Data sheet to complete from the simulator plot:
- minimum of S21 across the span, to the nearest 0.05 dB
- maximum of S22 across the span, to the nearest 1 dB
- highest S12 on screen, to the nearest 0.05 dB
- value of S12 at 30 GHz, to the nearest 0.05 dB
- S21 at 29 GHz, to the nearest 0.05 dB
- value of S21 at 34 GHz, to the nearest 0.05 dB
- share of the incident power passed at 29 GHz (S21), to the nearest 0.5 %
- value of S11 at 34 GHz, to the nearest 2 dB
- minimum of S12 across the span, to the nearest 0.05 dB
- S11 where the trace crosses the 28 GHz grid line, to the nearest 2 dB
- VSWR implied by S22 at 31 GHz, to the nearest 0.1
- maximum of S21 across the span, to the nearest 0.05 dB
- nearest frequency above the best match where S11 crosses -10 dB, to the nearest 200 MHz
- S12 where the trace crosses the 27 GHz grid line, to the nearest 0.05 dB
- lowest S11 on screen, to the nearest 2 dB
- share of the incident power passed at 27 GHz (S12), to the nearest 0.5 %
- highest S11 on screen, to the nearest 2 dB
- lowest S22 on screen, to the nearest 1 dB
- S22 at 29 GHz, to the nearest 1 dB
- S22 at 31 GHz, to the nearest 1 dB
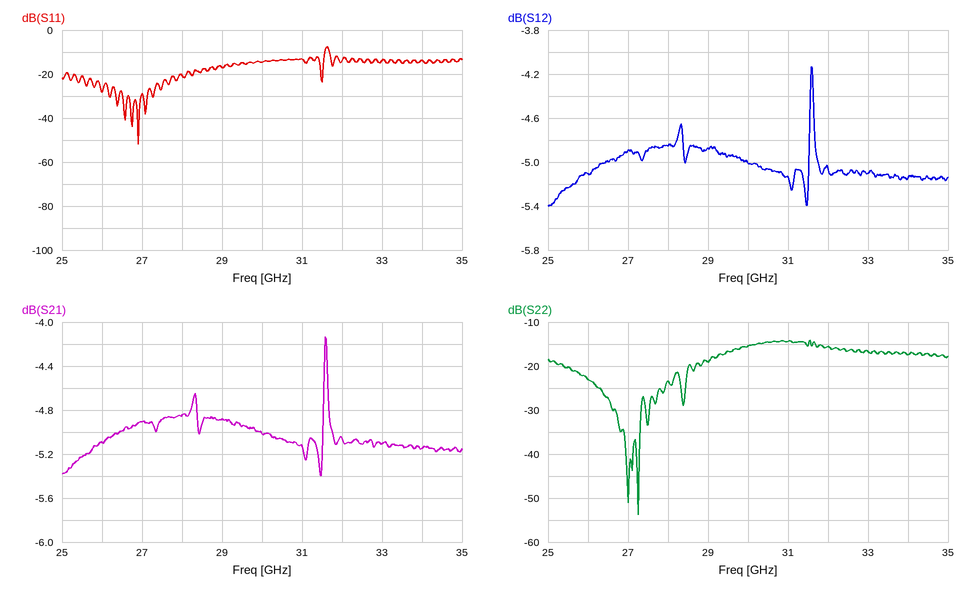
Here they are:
-5.40 dB
-14 dB
-4.15 dB
-5.00 dB
-4.90 dB
-5.15 dB
32.5 %
-14 dB
-5.40 dB
-20 dB
1.5
-4.15 dB
31.6 GHz
-4.90 dB
-52 dB
32.5 %
-8 dB
-54 dB
-19 dB
-14 dB
